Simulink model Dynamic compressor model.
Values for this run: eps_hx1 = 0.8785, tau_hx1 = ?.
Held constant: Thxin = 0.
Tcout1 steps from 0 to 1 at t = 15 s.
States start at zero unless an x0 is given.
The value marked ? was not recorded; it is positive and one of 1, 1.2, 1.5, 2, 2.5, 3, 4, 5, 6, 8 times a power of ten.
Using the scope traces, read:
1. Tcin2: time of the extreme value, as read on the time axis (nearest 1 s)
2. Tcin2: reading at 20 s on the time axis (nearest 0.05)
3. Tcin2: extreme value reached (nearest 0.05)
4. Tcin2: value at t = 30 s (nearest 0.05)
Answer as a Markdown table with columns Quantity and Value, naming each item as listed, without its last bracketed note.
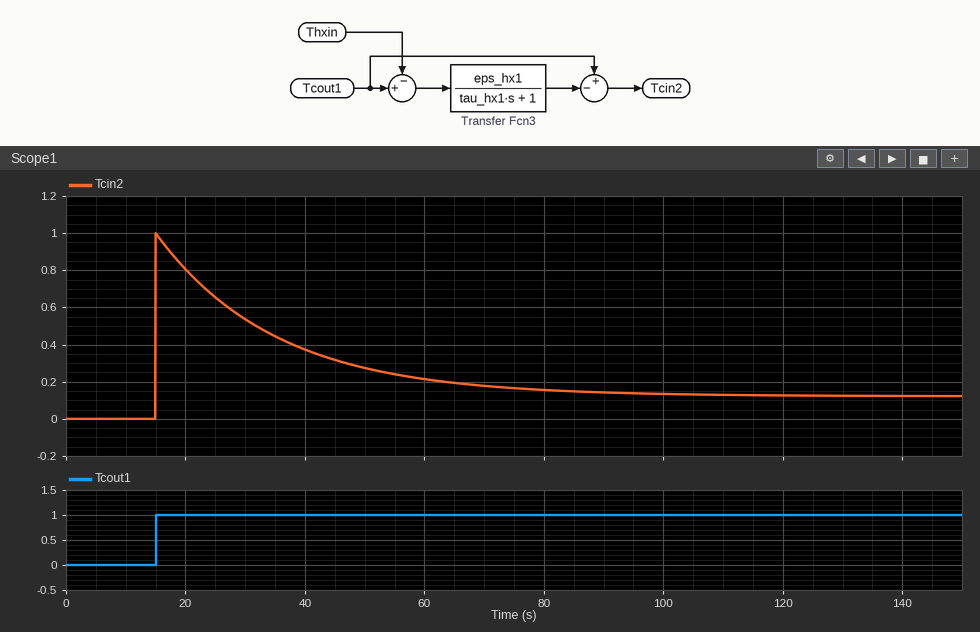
| Quantity | Value |
|---|---|
| Tcin2: time of the extreme value, as read on the time axis | 15 s |
| Tcin2: reading at 20 s on the time axis | 0.80 |
| Tcin2: extreme value reached | 1.00 |
| Tcin2: value at t = 30 s | 0.55 |
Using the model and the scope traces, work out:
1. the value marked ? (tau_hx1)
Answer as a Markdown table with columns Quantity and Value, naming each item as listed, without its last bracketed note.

| Quantity | Value |
|---|---|
| the value marked ? | 20 |
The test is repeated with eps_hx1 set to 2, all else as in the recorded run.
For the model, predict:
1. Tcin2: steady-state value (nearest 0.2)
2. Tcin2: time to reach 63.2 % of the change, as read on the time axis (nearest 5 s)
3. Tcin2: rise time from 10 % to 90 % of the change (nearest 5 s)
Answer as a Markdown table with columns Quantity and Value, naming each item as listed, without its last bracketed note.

| Quantity | Value |
|---|---|
| Tcin2: steady-state value | -1.0 |
| Tcin2: time to reach 63.2 % of the change, as read on the time axis | 50 s |
| Tcin2: rise time from 10 % to 90 % of the change | 45 s |
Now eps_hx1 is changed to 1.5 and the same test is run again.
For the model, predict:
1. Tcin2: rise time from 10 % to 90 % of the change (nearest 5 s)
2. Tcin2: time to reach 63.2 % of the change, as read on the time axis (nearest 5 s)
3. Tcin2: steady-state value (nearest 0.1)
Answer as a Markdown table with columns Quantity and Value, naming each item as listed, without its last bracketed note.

| Quantity | Value |
|---|---|
| Tcin2: rise time from 10 % to 90 % of the change | 45 s |
| Tcin2: time to reach 63.2 % of the change, as read on the time axis | 55 s |
| Tcin2: steady-state value | -0.5 |
